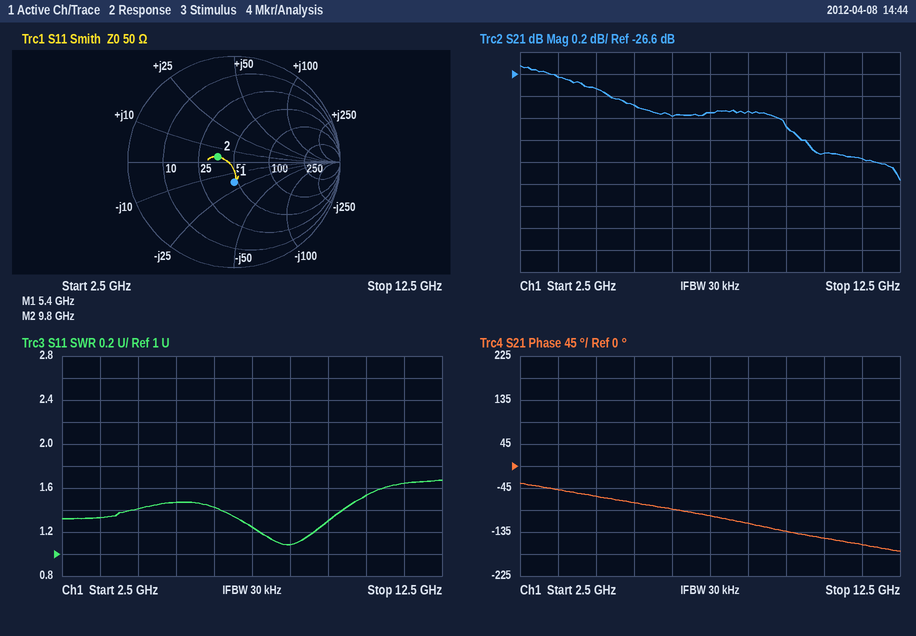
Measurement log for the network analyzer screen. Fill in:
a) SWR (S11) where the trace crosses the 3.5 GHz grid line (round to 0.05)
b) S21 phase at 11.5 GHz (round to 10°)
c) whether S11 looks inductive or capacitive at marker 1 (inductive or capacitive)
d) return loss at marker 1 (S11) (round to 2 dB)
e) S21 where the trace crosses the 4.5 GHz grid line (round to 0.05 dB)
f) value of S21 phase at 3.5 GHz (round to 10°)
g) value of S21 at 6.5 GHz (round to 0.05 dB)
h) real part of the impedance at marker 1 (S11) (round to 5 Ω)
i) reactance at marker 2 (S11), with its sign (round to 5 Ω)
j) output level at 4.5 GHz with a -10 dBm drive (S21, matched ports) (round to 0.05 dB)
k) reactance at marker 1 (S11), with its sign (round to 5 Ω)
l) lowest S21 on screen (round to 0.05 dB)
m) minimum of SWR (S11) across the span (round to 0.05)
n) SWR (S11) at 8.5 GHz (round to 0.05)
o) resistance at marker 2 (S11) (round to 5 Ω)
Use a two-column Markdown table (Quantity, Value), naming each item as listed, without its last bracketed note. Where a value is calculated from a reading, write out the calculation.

| Quantity | Value |
|---|---|
| SWR (S11) where the trace crosses the 3.5 GHz grid line | 1.35 |
| S21 phase at 11.5 GHz | -160° |
| whether S11 looks inductive or capacitive at marker 1 | capacitive |
| return loss at marker 1 (S11) | 14 dB |
| S21 where the trace crosses the 4.5 GHz grid line | -26.75 dB |
| value of S21 phase at 3.5 GHz | -50° |
| value of S21 at 6.5 GHz | -27.00 dB |
| real part of the impedance at marker 1 (S11) | 45 Ω |
| reactance at marker 2 (S11), with its sign | +5 Ω |
| output level at 4.5 GHz with a -10 dBm drive (S21, matched ports) | -10 dBm + (-26.75 dB) = -36.75 dBm |
| reactance at marker 1 (S11), with its sign | -20 Ω |
| lowest S21 on screen | -27.55 dB |
| minimum of SWR (S11) across the span | 1.10 |
| SWR (S11) at 8.5 GHz | 1.10 |
| resistance at marker 2 (S11) | 35 Ω |
